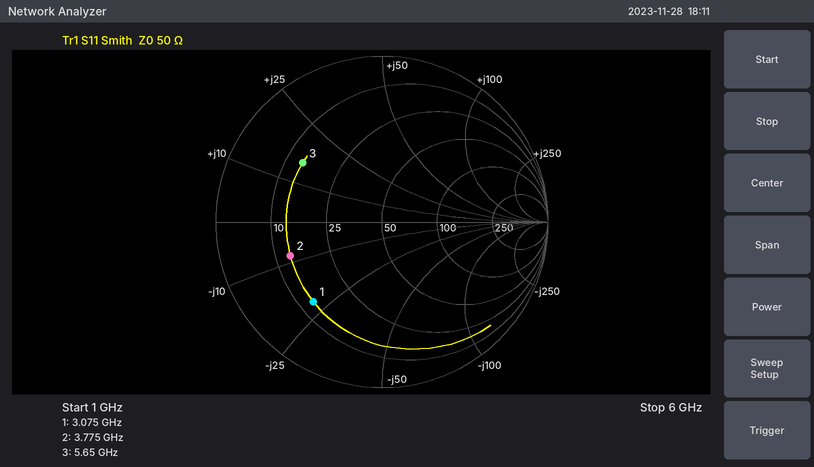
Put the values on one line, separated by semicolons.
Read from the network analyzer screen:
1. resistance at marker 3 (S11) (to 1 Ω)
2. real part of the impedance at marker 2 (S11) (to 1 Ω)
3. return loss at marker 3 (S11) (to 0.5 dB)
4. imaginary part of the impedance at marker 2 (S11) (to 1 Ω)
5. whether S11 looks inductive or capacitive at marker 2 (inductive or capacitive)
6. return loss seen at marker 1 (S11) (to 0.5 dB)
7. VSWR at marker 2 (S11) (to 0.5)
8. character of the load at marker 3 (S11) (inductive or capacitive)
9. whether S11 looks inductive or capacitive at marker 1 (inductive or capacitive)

14 Ω; 13 Ω; 4.5 dB; -8 Ω; capacitive; 4.0 dB; 4.0; inductive; capacitive
